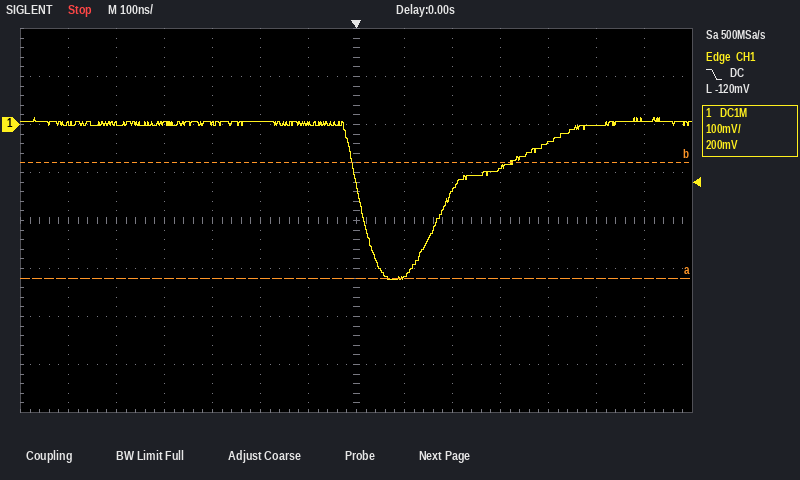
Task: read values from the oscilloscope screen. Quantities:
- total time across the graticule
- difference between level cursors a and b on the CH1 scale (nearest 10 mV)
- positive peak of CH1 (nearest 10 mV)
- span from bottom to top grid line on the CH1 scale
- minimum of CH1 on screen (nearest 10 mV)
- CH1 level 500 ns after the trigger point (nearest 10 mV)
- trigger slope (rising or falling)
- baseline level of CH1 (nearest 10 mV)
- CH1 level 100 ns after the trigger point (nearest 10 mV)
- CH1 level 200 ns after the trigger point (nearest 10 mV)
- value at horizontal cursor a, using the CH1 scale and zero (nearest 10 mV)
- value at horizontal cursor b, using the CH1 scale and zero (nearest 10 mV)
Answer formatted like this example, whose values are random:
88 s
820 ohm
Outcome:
1.4 µs
240 mV
10 mV
800 mV
-320 mV
0 mV
falling
0 mV
-320 mV
-140 mV
-320 mV
-80 mV
